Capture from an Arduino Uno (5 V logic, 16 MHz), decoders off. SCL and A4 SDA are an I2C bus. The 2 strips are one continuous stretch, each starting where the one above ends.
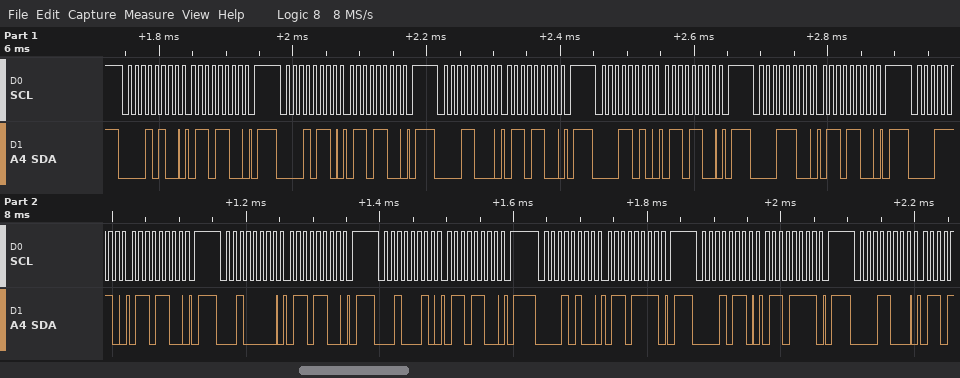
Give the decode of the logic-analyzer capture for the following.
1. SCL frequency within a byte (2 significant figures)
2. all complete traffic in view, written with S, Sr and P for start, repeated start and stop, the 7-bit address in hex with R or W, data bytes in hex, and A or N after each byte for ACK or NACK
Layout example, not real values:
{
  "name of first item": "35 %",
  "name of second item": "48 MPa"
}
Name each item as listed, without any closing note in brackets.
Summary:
{
  "SCL frequency within a byte": "100 kHz",
  "all complete traffic in view, written with S, Sr and P for start, repeated start and stop, the 7-bit address in hex with R or W, data bytes in hex, and A or N after each byte for ACK or NACK": "S 0AW A 6C A P S 0BW A 6C A P S 0CW A 6C A P S 0DW A 6C A P S 0EW A 6C A P S 0FW A 6C A P S 10W A 6C A P S 11W A 6C A P S 0AW A 6F A P S 0BW A 6F A P S 0CW A"
}
